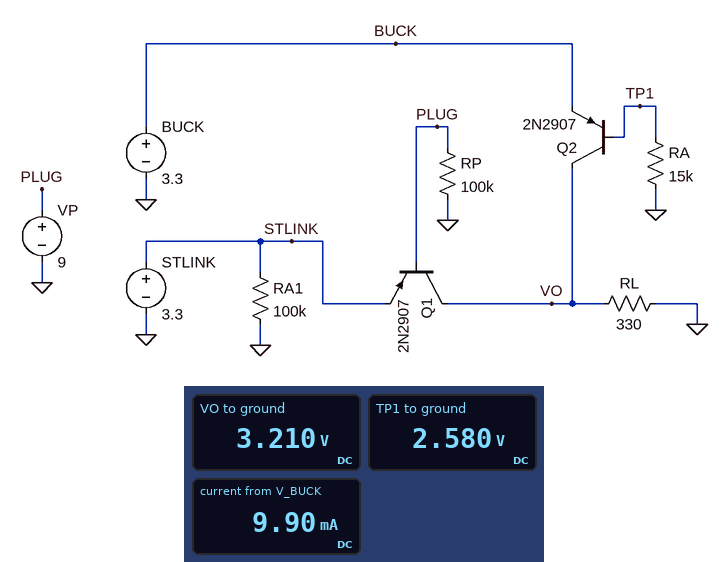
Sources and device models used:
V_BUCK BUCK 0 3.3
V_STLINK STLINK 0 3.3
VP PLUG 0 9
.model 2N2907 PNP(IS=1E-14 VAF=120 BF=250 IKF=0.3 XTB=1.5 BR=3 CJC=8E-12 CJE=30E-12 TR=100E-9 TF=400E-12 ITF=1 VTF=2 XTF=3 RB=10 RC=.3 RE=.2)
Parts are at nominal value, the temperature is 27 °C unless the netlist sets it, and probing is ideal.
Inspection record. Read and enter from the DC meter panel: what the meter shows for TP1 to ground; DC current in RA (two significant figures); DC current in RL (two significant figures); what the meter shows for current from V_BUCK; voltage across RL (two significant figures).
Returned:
2.580 V
170 µA
9.7 mA
9.90 mA
3.2 V
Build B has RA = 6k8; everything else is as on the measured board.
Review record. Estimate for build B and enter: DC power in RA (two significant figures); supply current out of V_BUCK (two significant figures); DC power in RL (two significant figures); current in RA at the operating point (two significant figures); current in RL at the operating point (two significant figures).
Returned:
980 µW
10 mA
32 mW
380 µA
9.8 mA
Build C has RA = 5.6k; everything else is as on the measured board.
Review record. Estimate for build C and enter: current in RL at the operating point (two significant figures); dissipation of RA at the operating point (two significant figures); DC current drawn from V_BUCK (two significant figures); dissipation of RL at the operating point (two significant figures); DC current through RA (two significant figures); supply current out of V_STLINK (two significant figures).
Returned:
9.8 mA
1.2 mW
10 mA
32 mW
460 µA
33 µA
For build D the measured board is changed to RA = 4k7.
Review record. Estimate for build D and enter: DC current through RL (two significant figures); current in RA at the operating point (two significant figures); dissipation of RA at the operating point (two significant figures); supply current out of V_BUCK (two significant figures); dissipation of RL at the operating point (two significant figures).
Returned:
9.8 mA
550 µA
1.4 mW
10 mA
32 mW
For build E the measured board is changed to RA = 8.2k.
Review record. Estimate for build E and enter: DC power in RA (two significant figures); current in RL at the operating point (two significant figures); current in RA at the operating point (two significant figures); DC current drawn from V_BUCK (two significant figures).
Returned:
810 µW
9.8 mA
310 µA
10 mA
